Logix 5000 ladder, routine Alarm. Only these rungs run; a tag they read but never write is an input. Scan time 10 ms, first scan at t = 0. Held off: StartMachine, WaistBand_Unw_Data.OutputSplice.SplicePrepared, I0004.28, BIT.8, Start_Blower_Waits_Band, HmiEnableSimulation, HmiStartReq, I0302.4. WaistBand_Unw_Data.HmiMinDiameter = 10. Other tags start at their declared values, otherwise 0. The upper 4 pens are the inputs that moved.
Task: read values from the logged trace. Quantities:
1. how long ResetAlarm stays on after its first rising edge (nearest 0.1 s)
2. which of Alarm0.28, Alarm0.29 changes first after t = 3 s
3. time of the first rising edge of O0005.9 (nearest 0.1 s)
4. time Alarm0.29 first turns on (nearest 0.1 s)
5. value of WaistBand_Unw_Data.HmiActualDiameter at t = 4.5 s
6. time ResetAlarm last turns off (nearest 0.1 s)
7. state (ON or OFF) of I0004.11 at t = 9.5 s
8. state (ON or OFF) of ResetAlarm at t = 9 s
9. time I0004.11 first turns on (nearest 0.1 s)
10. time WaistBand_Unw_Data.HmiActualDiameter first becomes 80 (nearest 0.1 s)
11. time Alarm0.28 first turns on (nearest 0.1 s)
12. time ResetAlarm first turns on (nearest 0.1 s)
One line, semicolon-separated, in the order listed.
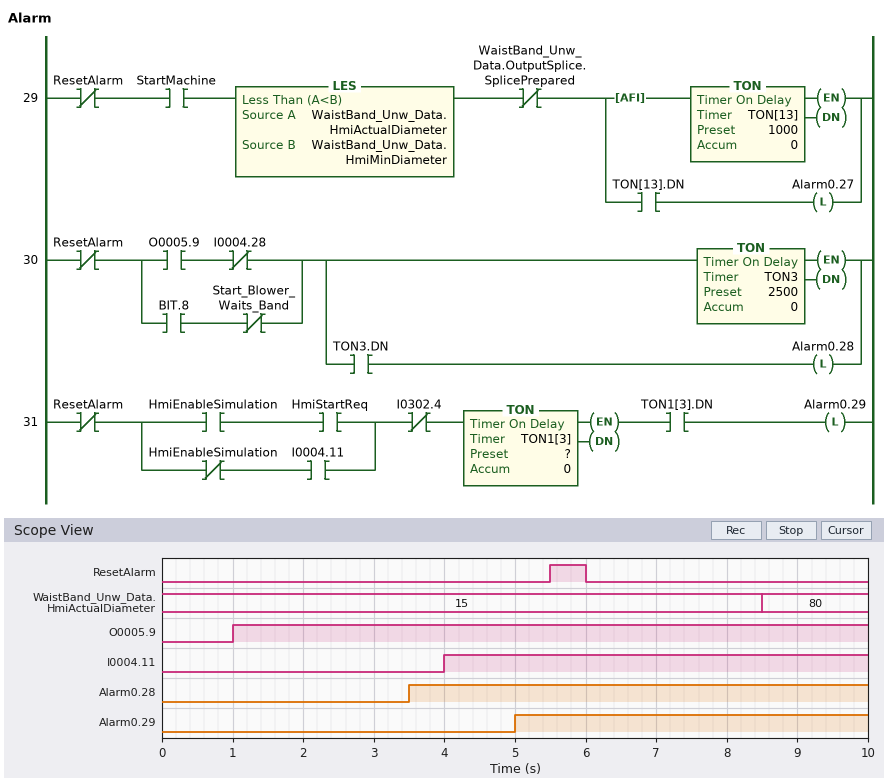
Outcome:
0.5 s; Alarm0.28; 1.0 s; 5.0 s; 15; 6.0 s; ON; OFF; 4.0 s; 8.5 s; 3.5 s; 5.5 s
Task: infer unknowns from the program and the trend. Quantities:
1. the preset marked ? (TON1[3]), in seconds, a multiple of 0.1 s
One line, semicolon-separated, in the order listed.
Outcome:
1.0 s
